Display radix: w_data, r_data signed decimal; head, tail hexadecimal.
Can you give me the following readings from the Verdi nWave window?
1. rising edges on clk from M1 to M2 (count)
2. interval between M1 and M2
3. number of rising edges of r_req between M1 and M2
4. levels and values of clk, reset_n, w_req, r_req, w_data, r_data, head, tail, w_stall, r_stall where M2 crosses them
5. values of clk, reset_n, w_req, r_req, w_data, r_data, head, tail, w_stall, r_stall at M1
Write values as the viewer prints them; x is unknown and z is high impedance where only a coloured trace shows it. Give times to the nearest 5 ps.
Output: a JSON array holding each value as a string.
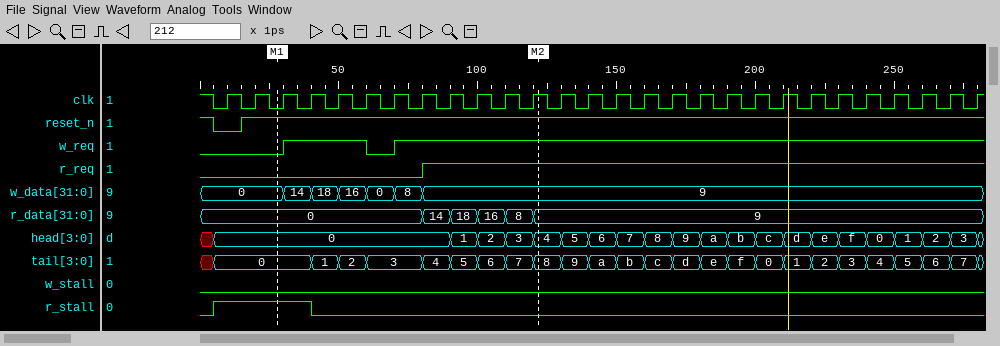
["10", "95 ps", "1", "clk=1, reset_n=1, w_req=1, r_req=1, w_data=9, r_data=9, head=4, tail=8, w_stall=0, r_stall=0", "clk=0, reset_n=1, w_req=0, r_req=0, w_data=0, r_data=0, head=0, tail=0, w_stall=0, r_stall=1"]
